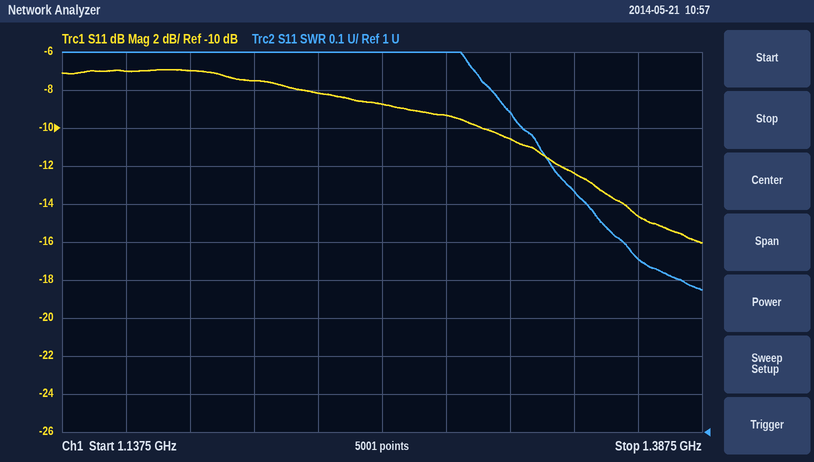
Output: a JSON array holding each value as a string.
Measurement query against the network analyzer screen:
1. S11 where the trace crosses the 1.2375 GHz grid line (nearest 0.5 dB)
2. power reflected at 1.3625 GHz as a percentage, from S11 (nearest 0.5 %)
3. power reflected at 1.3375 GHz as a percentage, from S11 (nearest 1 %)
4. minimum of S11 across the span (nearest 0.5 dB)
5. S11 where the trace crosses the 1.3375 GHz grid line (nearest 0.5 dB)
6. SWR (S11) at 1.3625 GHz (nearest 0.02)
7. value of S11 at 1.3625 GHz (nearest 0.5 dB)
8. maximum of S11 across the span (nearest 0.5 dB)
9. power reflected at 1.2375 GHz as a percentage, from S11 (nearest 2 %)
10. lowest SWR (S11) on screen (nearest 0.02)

["-8.0 dB", "3.5 %", "6 %", "-16.0 dB", "-12.5 dB", "1.46", "-14.5 dB", "-7.0 dB", "16 %", "1.38"]
